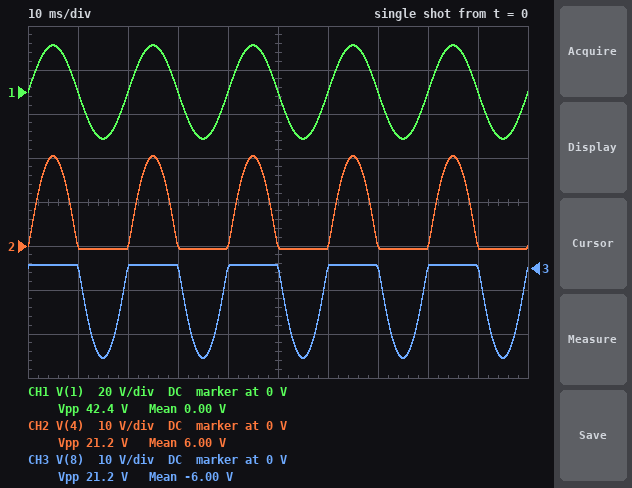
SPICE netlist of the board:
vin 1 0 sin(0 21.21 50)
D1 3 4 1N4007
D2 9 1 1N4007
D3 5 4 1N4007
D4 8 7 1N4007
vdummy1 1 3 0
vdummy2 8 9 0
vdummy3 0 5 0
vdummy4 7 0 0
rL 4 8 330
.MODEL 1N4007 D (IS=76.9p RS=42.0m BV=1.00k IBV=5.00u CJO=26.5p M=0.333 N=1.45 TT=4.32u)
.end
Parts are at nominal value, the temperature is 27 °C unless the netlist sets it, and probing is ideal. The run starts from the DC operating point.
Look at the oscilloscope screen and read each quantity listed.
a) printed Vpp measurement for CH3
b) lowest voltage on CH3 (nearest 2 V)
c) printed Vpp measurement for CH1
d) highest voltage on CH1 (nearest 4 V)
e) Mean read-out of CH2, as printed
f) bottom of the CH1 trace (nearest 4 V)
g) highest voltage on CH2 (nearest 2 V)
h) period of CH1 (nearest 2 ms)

21.2 V
-20 V
42.4 V
20 V
6.00 V
-20 V
20 V
20 ms
